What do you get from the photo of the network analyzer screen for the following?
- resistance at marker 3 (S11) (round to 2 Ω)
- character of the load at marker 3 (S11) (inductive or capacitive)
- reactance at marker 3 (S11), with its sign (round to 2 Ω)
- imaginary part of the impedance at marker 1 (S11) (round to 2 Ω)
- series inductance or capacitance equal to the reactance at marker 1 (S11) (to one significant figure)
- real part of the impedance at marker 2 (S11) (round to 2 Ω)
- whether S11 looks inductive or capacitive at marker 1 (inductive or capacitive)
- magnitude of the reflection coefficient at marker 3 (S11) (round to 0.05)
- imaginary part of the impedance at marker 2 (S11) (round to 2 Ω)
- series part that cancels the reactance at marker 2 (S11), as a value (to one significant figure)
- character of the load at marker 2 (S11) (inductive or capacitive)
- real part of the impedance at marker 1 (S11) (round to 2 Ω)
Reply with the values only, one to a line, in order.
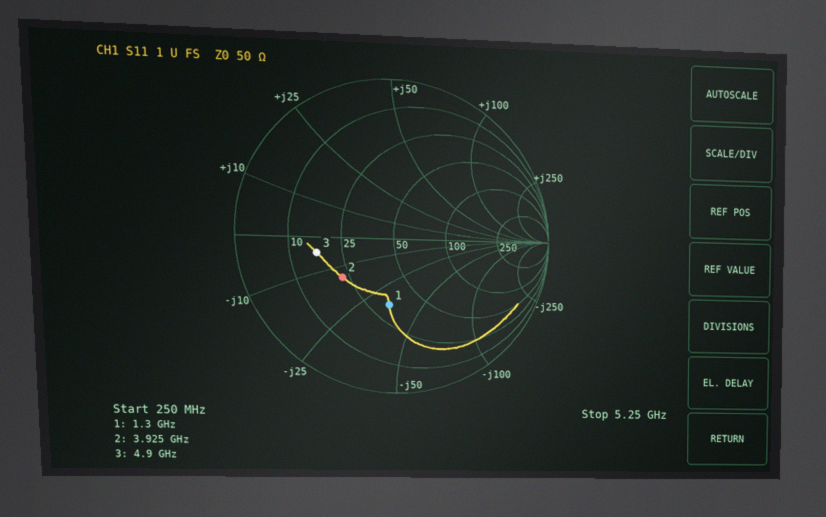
16 Ω
capacitive
-4 Ω
-34 Ω
4 pF
22 Ω
capacitive
0.50
-14 Ω
600 pH
capacitive
32 Ω
